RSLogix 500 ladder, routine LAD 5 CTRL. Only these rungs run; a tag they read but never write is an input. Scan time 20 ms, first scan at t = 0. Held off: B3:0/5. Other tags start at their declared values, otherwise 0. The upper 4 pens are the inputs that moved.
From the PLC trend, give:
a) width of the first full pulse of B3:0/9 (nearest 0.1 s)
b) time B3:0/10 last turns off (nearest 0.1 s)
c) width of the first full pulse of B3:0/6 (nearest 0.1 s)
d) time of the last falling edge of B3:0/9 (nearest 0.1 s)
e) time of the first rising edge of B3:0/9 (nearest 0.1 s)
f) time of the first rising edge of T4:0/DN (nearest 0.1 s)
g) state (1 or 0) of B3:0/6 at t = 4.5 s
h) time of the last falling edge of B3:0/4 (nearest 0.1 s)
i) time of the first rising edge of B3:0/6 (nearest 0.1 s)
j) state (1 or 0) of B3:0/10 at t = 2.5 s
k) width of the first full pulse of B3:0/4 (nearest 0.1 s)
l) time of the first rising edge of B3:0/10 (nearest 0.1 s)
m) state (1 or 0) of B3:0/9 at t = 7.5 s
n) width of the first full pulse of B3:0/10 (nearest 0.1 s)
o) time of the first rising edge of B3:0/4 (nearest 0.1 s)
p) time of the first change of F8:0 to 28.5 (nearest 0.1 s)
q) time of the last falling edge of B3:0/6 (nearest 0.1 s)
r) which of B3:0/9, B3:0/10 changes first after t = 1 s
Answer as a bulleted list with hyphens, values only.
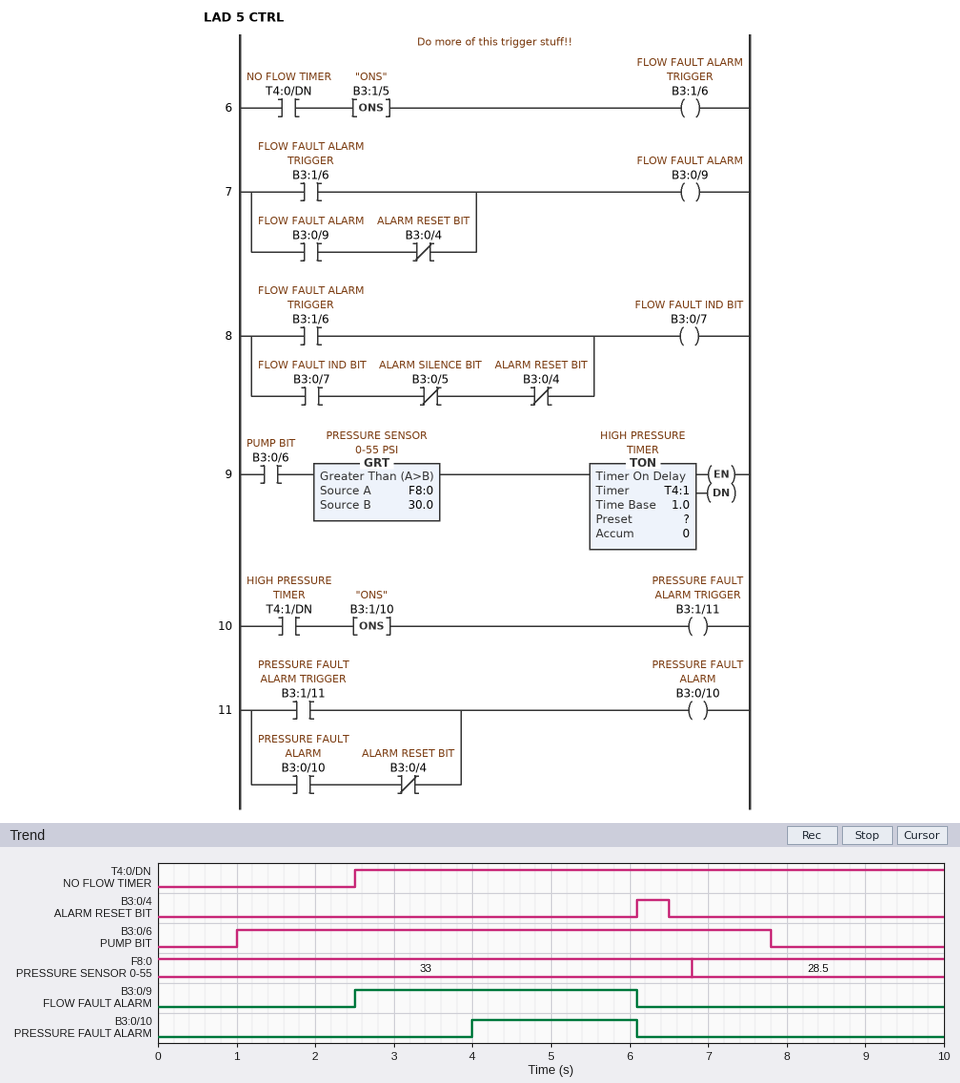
- 3.6 s
- 6.1 s
- 6.8 s
- 6.1 s
- 2.5 s
- 2.5 s
- 1
- 6.5 s
- 1.0 s
- 0
- 0.4 s
- 4.0 s
- 0
- 2.1 s
- 6.1 s
- 6.8 s
- 7.8 s
- B3:0/9
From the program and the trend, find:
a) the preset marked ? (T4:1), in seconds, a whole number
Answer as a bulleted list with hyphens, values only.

- 3 s
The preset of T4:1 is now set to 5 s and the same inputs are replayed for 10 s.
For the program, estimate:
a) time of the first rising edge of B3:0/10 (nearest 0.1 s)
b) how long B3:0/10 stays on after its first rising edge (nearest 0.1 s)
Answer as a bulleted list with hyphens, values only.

- 6.0 s
- 0.1 s
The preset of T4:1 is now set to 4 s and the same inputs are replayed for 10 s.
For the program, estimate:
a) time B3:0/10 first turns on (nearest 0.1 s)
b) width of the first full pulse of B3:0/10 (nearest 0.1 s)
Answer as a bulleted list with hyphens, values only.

- 5.0 s
- 1.1 s
